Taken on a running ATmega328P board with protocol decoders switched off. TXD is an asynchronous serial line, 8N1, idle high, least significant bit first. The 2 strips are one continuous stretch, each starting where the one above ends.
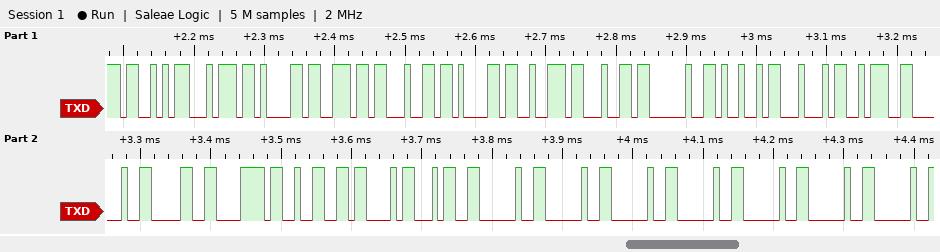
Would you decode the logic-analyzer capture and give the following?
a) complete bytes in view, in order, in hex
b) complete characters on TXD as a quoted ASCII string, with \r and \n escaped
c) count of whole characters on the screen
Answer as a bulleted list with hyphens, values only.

- 53 74 61 6E 64 61 72 64 20 49 44 3A 20 30 78 32 43 34 20 20 20 20 20 20 20
- "Standard ID: 0x2C4       "
- 25
